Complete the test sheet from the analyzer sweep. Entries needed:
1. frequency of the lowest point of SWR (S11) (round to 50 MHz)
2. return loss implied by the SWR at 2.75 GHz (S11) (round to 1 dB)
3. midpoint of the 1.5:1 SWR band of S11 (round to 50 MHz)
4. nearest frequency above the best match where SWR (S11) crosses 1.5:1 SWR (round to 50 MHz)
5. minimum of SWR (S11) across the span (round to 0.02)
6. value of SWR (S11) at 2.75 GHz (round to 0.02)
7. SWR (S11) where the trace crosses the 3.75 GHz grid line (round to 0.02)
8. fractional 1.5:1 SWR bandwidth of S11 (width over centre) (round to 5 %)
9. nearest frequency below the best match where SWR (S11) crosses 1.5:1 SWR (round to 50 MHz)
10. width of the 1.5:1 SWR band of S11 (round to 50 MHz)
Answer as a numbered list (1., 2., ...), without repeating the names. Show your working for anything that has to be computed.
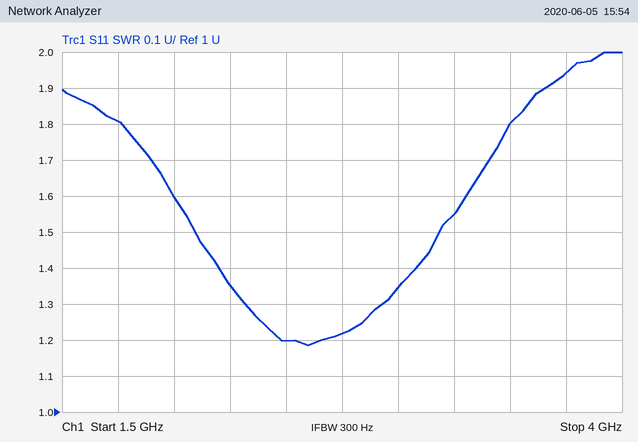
1. 2.60 GHz
2. −20 log10((1.22 − 1)/(1.22 + 1)) ≈ 20 dB
3. 2.65 GHz
4. 3.20 GHz
5. 1.18
6. 1.22
7. 1.94
8. 1.1 GHz / 2.65 GHz ≈ 41.5 %, so 40 % to the nearest 5 %
9. 2.10 GHz
10. 3.20 GHz − 2.10 GHz = 1.10 GHz
